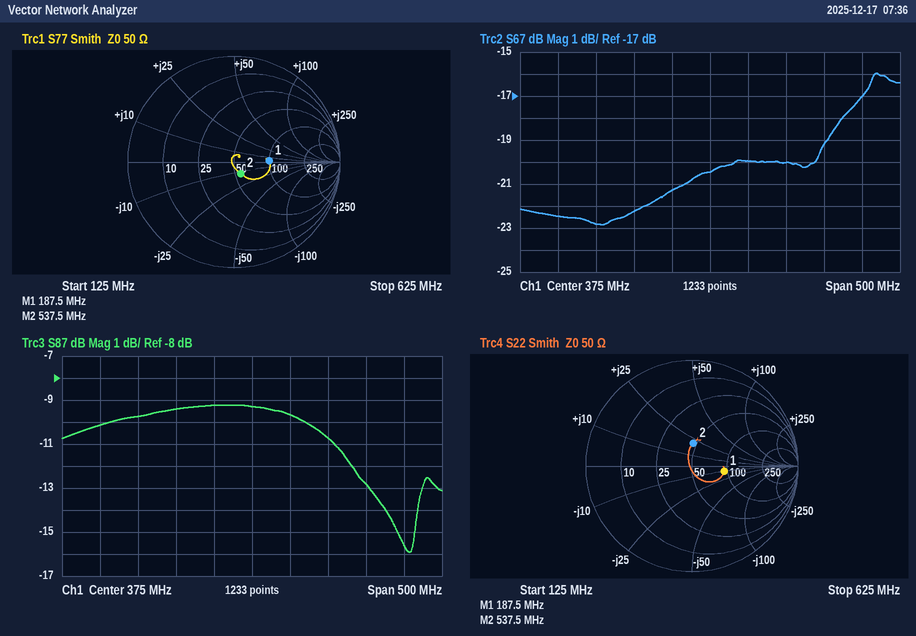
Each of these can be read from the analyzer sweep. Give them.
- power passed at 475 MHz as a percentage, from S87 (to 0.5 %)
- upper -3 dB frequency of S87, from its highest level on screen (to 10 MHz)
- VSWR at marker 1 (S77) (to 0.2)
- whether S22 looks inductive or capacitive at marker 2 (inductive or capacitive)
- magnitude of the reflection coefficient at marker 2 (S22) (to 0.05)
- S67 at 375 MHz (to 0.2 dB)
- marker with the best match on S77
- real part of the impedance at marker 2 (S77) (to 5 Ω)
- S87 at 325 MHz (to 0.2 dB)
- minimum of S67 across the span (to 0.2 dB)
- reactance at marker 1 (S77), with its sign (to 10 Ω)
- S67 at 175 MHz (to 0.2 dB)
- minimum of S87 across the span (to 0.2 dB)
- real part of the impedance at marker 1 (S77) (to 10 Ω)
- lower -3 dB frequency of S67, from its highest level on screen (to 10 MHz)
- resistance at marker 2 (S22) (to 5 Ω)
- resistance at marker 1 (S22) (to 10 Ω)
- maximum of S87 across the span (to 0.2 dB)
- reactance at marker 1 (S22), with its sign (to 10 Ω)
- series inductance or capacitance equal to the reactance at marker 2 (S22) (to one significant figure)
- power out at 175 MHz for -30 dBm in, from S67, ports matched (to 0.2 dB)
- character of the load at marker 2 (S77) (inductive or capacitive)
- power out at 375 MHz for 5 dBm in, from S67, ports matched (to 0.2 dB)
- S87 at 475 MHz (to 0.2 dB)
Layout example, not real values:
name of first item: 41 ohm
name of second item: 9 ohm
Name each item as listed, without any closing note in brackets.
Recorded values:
power passed at 475 MHz as a percentage, from S87: 8.5 %
upper -3 dB frequency of S87, from its highest level on screen: 510 MHz
VSWR at marker 1 (S77): 2.0
whether S22 looks inductive or capacitive at marker 2: inductive
magnitude of the reflection coefficient at marker 2 (S22): 0.20
S67 at 375 MHz: -20.4 dB
marker with the best match on S77: marker 2
real part of the impedance at marker 2 (S77): 55 Ω
S87 at 325 MHz: -9.2 dB
minimum of S67 across the span: -22.8 dB
reactance at marker 1 (S77), with its sign: 0 Ω
S67 at 175 MHz: -22.4 dB
minimum of S87 across the span: -16.0 dB
real part of the impedance at marker 1 (S77): 100 Ω
lower -3 dB frequency of S67, from its highest level on screen: 530 MHz
resistance at marker 2 (S22): 45 Ω
resistance at marker 1 (S22): 90 Ω
maximum of S87 across the span: -9.2 dB
reactance at marker 1 (S22), with its sign: -10 Ω
series inductance or capacitance equal to the reactance at marker 2 (S22): 6 nH
power out at 175 MHz for -30 dBm in, from S67, ports matched: -52.4 dBm
character of the load at marker 2 (S77): capacitive
power out at 375 MHz for 5 dBm in, from S67, ports matched: -15.4 dBm
S87 at 475 MHz: -10.8 dB
